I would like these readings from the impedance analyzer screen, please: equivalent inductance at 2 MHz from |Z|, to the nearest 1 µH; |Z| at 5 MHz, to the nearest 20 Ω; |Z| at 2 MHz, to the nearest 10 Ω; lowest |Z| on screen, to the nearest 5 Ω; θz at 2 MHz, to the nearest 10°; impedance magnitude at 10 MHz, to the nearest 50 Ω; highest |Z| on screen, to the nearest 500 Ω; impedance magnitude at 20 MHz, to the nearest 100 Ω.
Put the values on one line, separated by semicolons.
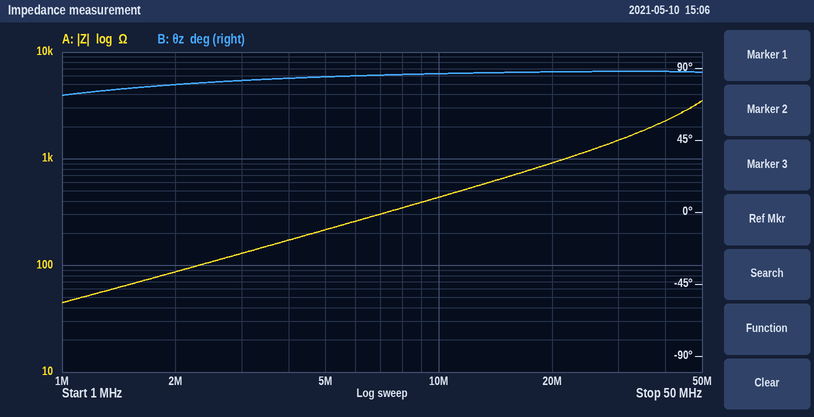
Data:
7 µH; 220 Ω; 90 Ω; 45 Ω; 80°; 450 Ω; 3.5 kΩ; 900 Ω
